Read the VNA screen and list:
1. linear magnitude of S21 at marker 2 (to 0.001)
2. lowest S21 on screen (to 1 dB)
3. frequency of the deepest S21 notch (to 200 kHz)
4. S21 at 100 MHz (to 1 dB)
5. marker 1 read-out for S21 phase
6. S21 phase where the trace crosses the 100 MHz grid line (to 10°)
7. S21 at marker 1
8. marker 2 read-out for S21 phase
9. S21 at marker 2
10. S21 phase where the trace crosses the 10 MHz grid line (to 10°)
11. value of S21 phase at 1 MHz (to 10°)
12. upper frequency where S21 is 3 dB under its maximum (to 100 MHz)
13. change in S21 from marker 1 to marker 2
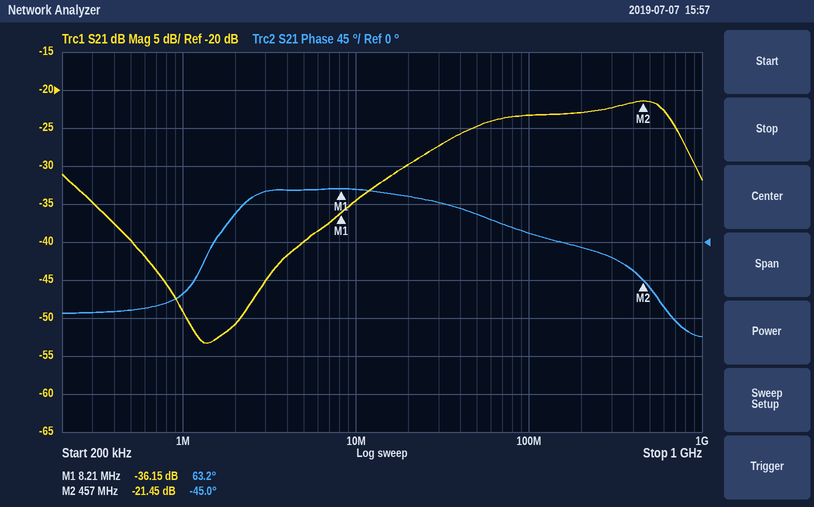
0.085
-53 dB
1.4 MHz
-23 dB
63.2°
10°
-36.15 dB
-45.0°
-21.45 dB
60°
-60°
700 MHz
14.70 dB
